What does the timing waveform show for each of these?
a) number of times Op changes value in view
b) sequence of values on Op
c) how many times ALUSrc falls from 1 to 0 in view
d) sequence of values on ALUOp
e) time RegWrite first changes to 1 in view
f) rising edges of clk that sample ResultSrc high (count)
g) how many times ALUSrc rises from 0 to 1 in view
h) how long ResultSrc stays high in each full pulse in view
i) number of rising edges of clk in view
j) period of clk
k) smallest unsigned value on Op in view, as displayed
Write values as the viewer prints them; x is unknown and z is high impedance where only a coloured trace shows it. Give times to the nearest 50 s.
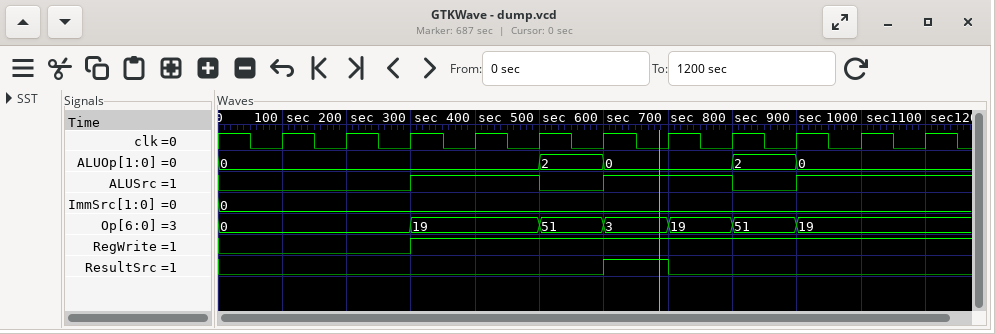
6
0, 19, 51, 3, 19, 51, 19
2
0, 2, 0, 2, 0
300 s
1
3
100 s
11
100 s
0
